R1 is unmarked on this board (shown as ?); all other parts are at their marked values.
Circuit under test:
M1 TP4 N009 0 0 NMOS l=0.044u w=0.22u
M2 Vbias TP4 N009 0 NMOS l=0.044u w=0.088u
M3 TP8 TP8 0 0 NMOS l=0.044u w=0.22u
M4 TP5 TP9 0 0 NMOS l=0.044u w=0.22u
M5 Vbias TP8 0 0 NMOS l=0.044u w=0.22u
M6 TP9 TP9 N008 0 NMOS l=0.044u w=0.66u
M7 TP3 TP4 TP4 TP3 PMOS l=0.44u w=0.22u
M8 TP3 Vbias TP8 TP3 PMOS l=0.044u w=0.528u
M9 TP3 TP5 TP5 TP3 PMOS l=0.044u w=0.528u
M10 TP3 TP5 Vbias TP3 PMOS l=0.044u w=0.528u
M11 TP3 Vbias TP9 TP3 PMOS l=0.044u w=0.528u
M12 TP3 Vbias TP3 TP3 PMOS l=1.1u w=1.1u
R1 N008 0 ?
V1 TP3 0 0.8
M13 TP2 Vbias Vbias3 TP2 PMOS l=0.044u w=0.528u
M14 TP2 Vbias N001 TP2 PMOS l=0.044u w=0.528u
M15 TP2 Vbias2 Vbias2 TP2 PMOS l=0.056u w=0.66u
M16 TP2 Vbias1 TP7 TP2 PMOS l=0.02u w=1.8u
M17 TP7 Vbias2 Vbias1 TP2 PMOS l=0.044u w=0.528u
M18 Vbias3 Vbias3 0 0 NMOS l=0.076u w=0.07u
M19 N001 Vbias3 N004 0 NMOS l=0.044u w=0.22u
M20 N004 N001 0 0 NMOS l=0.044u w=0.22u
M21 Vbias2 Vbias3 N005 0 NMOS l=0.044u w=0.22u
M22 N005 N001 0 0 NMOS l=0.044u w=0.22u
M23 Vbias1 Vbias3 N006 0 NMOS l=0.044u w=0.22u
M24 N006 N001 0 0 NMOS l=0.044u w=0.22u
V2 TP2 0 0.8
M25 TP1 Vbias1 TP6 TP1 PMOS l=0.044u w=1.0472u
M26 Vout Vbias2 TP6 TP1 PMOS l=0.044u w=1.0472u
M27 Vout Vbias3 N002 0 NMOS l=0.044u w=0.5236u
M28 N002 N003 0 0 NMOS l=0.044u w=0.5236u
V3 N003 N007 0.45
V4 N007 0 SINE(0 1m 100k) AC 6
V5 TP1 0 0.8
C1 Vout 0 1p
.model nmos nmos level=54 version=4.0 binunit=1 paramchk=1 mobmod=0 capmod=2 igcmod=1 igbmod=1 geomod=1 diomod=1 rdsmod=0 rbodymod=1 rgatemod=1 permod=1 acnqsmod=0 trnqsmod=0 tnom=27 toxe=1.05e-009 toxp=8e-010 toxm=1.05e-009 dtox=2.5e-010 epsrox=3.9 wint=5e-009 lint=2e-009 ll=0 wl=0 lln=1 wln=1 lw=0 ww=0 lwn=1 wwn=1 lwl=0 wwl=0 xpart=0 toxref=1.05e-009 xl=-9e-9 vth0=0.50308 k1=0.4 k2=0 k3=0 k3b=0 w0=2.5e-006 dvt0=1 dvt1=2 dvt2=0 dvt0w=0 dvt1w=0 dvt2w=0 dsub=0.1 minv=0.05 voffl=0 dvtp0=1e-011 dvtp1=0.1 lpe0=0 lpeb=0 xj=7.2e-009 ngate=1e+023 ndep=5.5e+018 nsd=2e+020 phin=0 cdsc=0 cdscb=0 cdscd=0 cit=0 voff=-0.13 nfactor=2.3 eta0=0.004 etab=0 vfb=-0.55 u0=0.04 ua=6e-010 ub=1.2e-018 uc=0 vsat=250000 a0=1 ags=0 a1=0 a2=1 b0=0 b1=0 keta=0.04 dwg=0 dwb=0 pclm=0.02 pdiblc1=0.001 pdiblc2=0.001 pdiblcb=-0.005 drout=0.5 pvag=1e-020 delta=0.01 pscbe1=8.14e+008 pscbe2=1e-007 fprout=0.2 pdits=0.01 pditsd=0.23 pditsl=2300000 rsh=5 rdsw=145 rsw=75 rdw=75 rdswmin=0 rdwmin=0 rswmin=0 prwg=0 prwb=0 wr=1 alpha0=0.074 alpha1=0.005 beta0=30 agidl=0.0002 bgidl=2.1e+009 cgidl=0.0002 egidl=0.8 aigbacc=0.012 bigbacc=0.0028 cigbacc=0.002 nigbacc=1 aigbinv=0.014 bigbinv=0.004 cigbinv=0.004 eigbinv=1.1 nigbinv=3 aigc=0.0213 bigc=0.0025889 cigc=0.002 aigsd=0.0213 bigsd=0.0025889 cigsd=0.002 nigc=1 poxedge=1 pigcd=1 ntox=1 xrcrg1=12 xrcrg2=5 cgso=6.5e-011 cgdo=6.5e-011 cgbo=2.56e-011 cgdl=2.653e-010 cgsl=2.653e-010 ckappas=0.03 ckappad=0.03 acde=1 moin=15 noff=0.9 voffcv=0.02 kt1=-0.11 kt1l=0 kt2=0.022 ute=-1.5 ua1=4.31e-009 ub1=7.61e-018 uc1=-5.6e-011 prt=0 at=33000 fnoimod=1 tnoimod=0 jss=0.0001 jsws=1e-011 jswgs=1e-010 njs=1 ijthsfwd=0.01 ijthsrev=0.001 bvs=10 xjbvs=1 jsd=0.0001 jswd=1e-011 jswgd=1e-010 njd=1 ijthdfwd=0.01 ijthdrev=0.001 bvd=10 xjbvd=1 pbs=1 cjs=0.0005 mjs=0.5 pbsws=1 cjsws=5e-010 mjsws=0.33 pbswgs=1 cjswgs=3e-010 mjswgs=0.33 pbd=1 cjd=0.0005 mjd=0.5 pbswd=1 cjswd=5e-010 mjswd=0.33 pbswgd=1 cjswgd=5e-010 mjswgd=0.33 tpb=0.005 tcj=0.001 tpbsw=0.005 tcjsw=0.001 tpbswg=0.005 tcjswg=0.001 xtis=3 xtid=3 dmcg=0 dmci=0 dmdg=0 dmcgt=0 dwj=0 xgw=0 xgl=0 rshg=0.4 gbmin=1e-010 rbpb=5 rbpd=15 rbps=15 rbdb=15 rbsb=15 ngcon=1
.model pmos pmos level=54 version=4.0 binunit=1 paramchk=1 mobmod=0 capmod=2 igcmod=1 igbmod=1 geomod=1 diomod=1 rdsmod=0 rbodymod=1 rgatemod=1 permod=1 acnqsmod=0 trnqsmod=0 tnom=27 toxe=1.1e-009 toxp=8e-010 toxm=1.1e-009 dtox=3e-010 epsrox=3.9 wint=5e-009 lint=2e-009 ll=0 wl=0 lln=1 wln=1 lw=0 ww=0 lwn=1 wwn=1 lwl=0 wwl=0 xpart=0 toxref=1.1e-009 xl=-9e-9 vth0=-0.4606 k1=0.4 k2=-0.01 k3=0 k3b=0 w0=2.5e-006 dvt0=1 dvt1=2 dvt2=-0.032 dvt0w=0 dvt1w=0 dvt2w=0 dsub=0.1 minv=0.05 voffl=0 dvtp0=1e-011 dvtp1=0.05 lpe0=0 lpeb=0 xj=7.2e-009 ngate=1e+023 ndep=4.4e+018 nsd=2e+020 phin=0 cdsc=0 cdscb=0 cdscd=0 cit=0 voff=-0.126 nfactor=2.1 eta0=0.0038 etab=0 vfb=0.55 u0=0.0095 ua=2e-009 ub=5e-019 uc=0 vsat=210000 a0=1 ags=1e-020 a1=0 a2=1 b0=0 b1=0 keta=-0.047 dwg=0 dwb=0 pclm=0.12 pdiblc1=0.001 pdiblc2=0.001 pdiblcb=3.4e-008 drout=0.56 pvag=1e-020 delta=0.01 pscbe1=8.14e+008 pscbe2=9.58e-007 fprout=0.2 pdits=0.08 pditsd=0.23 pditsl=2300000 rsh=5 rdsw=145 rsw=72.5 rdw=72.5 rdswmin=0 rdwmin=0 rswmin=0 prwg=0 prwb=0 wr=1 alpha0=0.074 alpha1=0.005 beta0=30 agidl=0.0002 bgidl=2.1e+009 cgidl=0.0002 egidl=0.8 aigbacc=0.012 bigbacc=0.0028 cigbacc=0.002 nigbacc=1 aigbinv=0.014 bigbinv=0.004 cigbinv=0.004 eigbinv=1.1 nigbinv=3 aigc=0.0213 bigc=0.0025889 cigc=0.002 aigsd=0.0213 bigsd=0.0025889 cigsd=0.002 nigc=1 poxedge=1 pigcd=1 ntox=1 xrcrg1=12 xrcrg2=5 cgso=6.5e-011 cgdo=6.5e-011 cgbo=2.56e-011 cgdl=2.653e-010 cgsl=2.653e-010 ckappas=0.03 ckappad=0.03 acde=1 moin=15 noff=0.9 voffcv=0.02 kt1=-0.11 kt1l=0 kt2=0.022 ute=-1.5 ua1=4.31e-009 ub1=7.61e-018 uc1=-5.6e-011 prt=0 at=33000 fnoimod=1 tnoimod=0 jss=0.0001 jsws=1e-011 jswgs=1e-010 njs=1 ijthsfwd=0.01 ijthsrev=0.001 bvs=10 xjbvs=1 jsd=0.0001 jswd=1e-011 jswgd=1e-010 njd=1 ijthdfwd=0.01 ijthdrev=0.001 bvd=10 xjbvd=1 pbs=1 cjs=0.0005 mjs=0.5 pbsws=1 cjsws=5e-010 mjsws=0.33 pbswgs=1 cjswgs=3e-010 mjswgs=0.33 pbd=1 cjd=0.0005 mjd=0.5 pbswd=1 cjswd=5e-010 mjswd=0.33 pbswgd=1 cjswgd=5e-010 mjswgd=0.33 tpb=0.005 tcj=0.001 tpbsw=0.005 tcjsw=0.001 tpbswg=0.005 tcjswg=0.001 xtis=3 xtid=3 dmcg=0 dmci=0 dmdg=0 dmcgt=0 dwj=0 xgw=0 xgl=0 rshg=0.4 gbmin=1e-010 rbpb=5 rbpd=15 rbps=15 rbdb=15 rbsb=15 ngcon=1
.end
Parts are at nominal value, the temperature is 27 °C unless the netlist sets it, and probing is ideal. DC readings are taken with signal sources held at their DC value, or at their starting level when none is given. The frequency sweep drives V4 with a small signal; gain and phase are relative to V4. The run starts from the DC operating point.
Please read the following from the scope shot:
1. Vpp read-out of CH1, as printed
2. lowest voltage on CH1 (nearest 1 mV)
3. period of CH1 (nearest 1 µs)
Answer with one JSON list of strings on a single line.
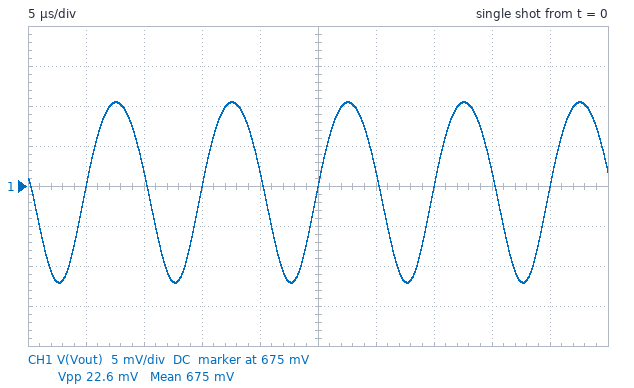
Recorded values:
["22.6 mV", "663 mV", "10 µs"]
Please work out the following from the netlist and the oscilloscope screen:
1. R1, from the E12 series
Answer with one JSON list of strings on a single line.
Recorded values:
["4.7 kΩ"]
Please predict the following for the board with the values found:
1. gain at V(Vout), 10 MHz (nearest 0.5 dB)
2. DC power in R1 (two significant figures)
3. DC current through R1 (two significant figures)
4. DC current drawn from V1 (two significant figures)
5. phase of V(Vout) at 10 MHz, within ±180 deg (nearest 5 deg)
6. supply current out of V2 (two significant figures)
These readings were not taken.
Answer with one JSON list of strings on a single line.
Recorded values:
["2.0 dB", "640 nW", "12 µA", "44 µA", "95 deg", "43 µA"]
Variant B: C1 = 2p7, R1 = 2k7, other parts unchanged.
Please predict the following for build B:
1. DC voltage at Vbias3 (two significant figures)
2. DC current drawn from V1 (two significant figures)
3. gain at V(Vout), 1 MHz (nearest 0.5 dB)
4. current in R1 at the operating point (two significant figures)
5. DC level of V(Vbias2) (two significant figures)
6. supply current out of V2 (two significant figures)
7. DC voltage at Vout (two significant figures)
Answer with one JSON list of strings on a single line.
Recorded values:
["750 mV", "88 µA", "-4.5 dB", "24 µA", "180 mV", "74 µA", "770 mV"]
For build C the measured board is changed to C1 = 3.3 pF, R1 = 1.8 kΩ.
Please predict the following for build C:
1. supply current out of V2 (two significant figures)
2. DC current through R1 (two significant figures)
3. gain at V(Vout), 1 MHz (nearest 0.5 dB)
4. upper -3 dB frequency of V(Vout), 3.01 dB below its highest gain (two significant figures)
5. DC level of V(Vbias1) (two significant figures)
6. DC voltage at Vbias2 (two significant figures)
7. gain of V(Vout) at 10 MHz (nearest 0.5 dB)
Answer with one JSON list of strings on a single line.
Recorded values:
["85 µA", "32 µA", "-6.0 dB", "8.0 MHz", "200 mV", "170 mV", "-10.0 dB"]
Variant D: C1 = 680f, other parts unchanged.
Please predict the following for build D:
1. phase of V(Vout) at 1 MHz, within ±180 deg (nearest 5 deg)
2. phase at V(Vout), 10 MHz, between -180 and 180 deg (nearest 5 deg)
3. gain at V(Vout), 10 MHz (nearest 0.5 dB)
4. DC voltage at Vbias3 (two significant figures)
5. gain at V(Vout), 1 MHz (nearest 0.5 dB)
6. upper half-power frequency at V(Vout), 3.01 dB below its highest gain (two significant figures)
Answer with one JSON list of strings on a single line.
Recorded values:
["150 deg", "100 deg", "5.5 dB", "710 mV", "19.5 dB", "1.7 MHz"]
